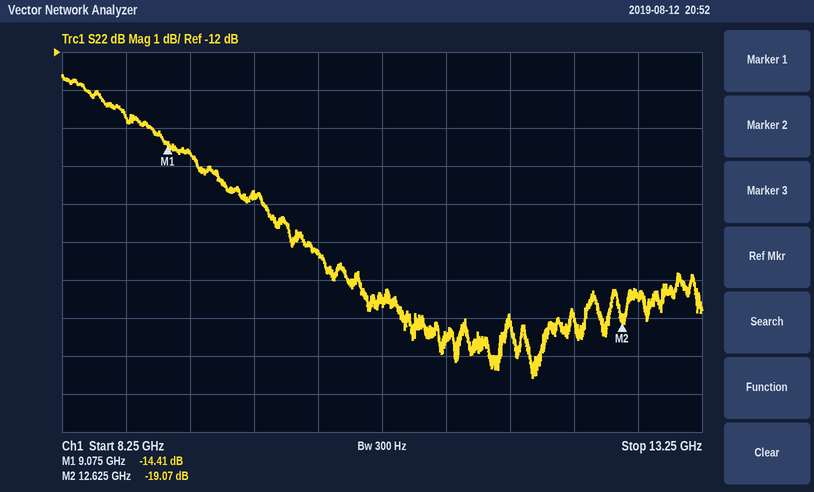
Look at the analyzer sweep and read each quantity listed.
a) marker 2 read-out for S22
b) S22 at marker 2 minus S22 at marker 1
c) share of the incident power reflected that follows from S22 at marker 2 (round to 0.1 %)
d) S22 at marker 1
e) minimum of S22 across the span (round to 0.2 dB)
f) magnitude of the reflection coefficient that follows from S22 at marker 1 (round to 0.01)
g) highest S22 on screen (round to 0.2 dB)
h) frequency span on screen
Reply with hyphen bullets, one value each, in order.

- -19.07 dB
- -4.66 dB
- 1.2 %
- -14.41 dB
- -20.6 dB
- 0.19
- -12.6 dB
- 5 GHz
